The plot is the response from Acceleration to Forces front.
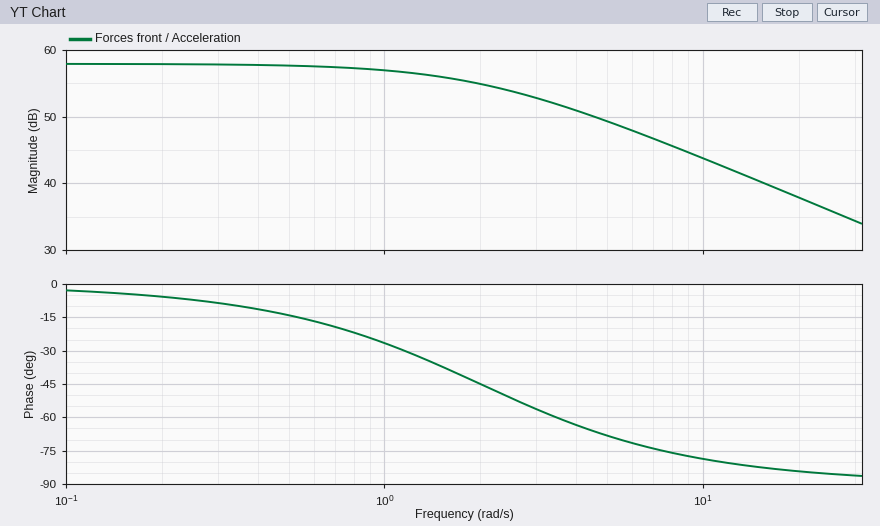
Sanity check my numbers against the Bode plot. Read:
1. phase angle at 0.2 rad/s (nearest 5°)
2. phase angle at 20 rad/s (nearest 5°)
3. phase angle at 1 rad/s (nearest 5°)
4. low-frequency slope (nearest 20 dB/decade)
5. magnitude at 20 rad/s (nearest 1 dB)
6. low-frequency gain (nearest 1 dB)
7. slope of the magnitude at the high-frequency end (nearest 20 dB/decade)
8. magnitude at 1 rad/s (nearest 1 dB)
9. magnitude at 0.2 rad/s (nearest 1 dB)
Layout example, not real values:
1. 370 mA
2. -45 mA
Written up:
1. -5°
2. -85°
3. -25°
4. 0 dB/decade
5. 38 dB
6. 58 dB
7. -20 dB/decade
8. 57 dB
9. 58 dB
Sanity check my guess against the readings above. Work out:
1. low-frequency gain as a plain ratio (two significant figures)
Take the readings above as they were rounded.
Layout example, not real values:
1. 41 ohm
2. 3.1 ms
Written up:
1. 790
